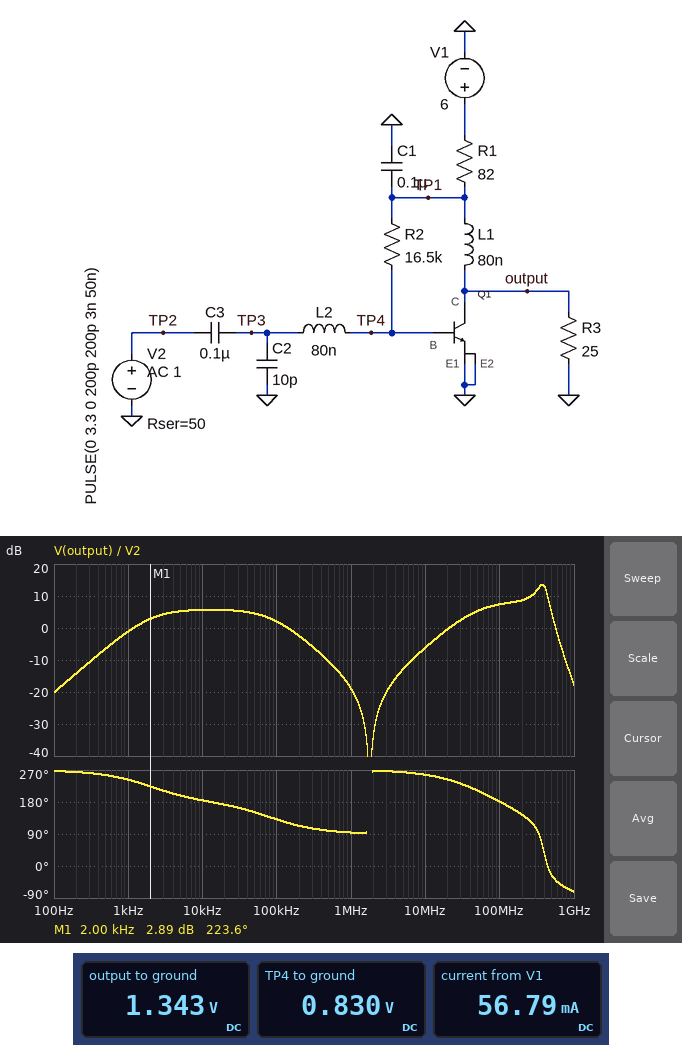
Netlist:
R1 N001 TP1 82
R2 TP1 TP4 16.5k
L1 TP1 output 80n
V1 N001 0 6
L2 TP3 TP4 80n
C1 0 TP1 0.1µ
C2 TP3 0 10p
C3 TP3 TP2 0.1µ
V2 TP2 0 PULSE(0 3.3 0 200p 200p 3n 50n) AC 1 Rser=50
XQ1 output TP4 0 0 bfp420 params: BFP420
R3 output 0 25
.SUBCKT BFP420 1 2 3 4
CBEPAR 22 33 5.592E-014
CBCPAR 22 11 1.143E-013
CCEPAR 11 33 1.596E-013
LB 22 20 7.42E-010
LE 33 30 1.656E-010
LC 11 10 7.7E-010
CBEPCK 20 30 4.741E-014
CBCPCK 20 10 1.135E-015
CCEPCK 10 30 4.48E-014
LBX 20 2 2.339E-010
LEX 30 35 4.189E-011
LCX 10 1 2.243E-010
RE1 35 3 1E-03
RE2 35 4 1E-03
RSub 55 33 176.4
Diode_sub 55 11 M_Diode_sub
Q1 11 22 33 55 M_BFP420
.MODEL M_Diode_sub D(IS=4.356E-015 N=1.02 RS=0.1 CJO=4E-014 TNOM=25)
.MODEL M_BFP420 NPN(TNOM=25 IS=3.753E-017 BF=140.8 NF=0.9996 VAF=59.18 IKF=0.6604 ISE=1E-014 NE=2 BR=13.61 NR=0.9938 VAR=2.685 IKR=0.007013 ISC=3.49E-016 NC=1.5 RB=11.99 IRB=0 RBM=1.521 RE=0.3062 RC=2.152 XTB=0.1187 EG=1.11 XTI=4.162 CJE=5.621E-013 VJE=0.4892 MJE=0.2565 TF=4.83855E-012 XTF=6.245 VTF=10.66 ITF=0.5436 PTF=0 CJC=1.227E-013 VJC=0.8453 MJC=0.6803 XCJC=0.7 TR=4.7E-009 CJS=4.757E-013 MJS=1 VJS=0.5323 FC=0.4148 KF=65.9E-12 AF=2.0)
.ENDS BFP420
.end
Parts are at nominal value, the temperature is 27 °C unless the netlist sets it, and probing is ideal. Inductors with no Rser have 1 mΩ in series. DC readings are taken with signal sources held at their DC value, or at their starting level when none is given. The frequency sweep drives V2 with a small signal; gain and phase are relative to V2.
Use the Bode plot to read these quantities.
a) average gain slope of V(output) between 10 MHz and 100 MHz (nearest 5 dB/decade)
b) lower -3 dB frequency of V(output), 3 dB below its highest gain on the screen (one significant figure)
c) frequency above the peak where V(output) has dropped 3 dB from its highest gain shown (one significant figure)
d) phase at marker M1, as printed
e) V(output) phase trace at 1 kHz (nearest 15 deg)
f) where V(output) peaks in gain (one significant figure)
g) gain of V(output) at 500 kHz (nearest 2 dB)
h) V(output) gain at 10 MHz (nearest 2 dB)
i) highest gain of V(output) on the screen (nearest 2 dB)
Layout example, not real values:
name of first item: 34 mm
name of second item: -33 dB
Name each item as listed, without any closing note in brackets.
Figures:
average gain slope of V(output) between 10 MHz and 100 MHz: 15 dB/decade
lower -3 dB frequency of V(output), 3 dB below its highest gain on the screen: 300 MHz
frequency above the peak where V(output) has dropped 3 dB from its highest gain shown: 400 MHz
phase at marker M1, as printed: 223.6 deg
V(output) phase trace at 1 kHz: 240 deg
where V(output) peaks in gain: 400 MHz
gain of V(output) at 500 kHz: -10 dB
V(output) gain at 10 MHz: -6 dB
highest gain of V(output) on the screen: 14 dB
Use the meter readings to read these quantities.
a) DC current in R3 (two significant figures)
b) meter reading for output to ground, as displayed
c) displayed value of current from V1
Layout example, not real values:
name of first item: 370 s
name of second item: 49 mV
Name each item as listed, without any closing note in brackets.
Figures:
DC current in R3: 54 mA
meter reading for output to ground, as displayed: 1.343 V
displayed value of current from V1: 56.79 mA
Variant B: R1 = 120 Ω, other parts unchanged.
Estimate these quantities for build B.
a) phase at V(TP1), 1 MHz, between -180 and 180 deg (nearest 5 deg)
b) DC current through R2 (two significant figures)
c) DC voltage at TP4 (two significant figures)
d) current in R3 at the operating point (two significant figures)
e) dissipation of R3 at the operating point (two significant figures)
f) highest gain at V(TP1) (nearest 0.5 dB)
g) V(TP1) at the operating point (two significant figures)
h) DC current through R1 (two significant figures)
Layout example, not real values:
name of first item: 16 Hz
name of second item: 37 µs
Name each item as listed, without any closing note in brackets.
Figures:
phase at V(TP1), 1 MHz, between -180 and 180 deg: 95 deg
DC current through R2: 12 µA
DC voltage at TP4: 810 mV
current in R3 at the operating point: 40 mA
dissipation of R3 at the operating point: 41 mW
highest gain at V(TP1): -1.0 dB
V(TP1) at the operating point: 1.0 V
DC current through R1: 42 mA
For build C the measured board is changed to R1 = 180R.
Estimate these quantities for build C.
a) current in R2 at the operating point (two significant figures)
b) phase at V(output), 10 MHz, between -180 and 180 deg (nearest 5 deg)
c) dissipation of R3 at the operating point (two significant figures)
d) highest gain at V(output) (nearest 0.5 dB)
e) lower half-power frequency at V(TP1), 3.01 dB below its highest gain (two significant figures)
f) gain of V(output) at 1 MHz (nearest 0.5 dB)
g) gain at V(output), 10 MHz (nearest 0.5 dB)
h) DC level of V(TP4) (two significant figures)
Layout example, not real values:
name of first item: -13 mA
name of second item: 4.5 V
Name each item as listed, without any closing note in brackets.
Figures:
current in R2 at the operating point: 510 nA
phase at V(output), 10 MHz, between -180 and 180 deg: -105 deg
dissipation of R3 at the operating point: 21 mW
highest gain at V(output): -11.5 dB
lower half-power frequency at V(TP1), 3.01 dB below its highest gain: 130 Hz
gain of V(output) at 1 MHz: -54.0 dB
gain at V(output), 10 MHz: -40.5 dB
DC level of V(TP4): 720 mV
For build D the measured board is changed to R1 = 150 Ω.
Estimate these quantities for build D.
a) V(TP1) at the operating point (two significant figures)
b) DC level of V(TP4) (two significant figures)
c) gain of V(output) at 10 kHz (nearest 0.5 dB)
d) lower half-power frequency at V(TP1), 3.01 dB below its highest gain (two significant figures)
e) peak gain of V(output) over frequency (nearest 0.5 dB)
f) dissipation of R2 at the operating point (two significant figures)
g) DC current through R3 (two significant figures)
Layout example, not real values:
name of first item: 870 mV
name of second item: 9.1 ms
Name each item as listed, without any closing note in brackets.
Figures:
V(TP1) at the operating point: 850 mV
DC level of V(TP4): 780 mV
gain of V(output) at 10 kHz: -9.5 dB
lower half-power frequency at V(TP1), 3.01 dB below its highest gain: 380 Hz
peak gain of V(output) over frequency: 3.5 dB
dissipation of R2 at the operating point: 300 nW
DC current through R3: 34 mA
